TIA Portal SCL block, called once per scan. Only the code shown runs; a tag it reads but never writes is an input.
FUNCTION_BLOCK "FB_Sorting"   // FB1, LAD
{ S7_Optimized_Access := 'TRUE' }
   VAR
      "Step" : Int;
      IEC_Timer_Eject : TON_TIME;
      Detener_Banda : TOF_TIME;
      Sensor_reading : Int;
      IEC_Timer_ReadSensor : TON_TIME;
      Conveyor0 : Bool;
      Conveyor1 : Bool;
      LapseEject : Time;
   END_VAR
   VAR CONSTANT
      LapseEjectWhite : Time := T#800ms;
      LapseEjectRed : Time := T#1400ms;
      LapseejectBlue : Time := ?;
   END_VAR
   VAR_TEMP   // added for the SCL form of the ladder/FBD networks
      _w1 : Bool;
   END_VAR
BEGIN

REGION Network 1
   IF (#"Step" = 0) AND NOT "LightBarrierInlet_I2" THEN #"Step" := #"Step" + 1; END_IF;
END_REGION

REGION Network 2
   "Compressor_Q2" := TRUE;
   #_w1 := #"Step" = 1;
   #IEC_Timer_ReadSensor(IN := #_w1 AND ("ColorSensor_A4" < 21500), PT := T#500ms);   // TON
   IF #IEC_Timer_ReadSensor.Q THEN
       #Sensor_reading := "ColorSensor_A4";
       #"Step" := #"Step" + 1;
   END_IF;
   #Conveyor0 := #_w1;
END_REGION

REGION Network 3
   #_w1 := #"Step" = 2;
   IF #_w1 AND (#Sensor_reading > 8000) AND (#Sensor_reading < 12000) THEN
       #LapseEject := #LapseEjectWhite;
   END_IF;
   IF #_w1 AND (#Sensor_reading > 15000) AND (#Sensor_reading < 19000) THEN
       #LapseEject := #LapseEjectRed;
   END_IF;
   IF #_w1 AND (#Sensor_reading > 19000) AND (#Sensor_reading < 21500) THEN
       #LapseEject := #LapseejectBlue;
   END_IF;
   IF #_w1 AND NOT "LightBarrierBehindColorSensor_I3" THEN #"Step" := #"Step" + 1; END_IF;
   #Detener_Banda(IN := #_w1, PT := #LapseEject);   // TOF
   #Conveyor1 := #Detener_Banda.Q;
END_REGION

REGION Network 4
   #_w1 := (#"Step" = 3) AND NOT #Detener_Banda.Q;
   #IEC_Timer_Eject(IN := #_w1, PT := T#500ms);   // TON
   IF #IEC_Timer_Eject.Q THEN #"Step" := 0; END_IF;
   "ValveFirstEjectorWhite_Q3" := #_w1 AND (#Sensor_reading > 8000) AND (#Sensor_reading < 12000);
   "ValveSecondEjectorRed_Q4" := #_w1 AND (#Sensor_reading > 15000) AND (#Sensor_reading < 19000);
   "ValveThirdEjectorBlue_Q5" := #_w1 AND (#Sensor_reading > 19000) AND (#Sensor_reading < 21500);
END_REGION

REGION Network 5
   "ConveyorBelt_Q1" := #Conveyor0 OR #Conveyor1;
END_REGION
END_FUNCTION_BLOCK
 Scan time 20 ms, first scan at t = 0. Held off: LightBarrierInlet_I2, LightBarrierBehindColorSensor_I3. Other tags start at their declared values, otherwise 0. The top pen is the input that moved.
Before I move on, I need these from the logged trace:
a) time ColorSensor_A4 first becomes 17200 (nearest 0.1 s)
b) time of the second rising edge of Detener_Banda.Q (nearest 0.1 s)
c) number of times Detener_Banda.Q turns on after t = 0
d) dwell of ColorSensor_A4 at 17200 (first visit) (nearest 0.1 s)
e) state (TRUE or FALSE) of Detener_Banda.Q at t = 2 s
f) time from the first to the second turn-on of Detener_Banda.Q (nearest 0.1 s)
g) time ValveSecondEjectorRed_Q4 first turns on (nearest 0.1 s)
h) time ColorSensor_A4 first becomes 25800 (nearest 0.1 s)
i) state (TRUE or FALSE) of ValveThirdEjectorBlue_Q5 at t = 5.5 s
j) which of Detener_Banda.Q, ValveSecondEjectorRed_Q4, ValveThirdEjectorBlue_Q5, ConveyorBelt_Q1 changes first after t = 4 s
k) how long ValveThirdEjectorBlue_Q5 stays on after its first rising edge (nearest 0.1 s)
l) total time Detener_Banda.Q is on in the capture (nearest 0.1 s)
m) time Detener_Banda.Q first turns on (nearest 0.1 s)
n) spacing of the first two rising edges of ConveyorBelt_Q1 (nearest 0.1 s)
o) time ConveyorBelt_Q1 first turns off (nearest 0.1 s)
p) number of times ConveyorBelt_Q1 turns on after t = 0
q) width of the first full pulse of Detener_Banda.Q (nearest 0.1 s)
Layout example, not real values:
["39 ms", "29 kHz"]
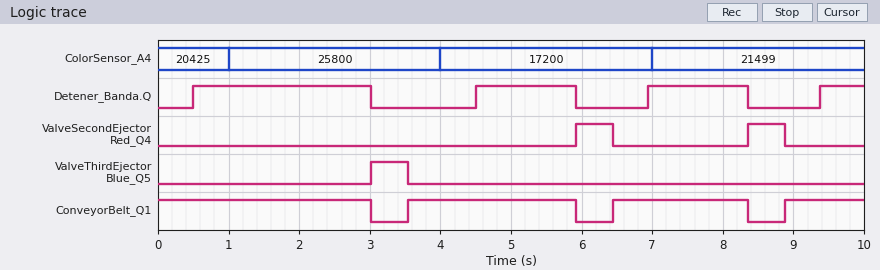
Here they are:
["4.0 s", "4.5 s", "4", "3.0 s", "TRUE", "4.0 s", "5.9 s", "1.0 s", "FALSE", "Detener_Banda.Q", "0.5 s", "6.0 s", "0.5 s", "2.9 s", "3.0 s", "3", "2.5 s"]
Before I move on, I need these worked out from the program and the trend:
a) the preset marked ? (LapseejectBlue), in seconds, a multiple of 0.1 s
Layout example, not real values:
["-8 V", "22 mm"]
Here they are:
["2.5 s"]
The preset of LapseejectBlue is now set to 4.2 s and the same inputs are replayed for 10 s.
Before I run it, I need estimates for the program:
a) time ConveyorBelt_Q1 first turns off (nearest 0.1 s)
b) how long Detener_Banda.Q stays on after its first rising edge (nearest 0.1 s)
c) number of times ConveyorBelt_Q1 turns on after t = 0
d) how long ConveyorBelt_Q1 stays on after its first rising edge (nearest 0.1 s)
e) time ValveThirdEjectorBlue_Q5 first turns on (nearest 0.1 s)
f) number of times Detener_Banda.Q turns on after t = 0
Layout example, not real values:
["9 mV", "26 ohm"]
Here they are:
["4.7 s", "4.2 s", "2", "1.9 s", "4.7 s", "3"]
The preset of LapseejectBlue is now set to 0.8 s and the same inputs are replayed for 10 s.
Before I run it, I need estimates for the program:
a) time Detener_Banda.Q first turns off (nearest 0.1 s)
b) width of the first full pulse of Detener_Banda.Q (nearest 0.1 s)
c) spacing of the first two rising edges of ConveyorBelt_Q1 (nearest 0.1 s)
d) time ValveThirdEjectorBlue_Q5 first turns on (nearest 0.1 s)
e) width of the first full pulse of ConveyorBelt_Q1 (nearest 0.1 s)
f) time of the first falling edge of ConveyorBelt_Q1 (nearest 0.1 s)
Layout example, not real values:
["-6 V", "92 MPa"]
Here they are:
["1.3 s", "0.8 s", "4.6 s", "1.3 s", "4.1 s", "1.3 s"]
